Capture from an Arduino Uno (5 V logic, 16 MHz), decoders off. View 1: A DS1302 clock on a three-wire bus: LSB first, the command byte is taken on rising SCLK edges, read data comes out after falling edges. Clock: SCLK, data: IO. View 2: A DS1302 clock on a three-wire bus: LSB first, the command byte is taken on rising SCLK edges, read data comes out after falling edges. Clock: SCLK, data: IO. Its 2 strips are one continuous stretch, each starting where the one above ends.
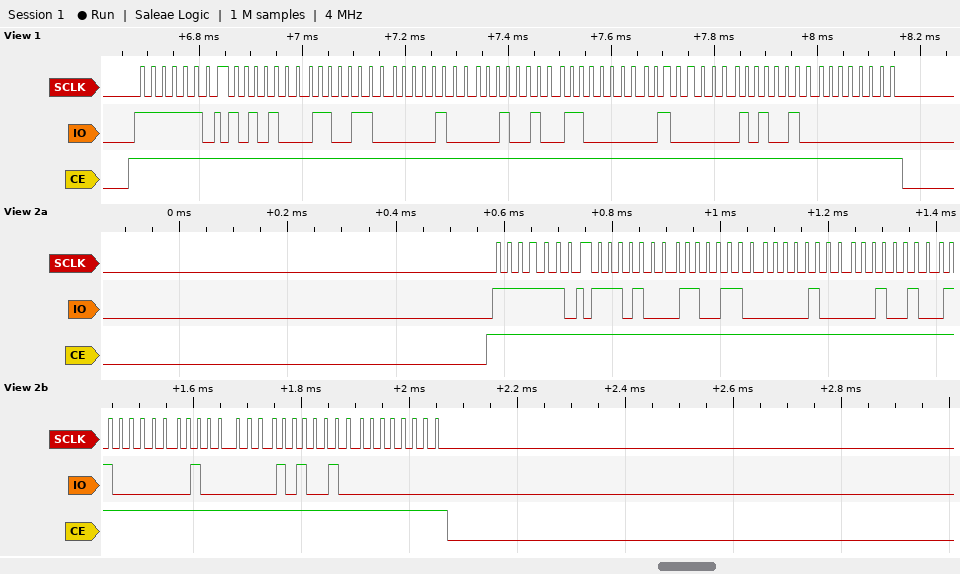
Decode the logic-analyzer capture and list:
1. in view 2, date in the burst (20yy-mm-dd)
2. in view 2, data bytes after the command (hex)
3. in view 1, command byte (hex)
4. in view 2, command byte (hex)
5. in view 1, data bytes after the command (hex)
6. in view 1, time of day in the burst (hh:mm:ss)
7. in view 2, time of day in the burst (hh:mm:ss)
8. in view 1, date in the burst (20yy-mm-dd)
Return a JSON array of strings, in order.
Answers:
["2025-03-24", "17 33 10 24 03 02 25 00", "0xBF", "0xBF", "15 33 10 24 03 02 25 00", "10:33:15", "10:33:17", "2025-03-24"]
